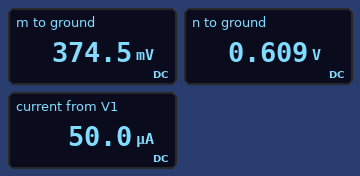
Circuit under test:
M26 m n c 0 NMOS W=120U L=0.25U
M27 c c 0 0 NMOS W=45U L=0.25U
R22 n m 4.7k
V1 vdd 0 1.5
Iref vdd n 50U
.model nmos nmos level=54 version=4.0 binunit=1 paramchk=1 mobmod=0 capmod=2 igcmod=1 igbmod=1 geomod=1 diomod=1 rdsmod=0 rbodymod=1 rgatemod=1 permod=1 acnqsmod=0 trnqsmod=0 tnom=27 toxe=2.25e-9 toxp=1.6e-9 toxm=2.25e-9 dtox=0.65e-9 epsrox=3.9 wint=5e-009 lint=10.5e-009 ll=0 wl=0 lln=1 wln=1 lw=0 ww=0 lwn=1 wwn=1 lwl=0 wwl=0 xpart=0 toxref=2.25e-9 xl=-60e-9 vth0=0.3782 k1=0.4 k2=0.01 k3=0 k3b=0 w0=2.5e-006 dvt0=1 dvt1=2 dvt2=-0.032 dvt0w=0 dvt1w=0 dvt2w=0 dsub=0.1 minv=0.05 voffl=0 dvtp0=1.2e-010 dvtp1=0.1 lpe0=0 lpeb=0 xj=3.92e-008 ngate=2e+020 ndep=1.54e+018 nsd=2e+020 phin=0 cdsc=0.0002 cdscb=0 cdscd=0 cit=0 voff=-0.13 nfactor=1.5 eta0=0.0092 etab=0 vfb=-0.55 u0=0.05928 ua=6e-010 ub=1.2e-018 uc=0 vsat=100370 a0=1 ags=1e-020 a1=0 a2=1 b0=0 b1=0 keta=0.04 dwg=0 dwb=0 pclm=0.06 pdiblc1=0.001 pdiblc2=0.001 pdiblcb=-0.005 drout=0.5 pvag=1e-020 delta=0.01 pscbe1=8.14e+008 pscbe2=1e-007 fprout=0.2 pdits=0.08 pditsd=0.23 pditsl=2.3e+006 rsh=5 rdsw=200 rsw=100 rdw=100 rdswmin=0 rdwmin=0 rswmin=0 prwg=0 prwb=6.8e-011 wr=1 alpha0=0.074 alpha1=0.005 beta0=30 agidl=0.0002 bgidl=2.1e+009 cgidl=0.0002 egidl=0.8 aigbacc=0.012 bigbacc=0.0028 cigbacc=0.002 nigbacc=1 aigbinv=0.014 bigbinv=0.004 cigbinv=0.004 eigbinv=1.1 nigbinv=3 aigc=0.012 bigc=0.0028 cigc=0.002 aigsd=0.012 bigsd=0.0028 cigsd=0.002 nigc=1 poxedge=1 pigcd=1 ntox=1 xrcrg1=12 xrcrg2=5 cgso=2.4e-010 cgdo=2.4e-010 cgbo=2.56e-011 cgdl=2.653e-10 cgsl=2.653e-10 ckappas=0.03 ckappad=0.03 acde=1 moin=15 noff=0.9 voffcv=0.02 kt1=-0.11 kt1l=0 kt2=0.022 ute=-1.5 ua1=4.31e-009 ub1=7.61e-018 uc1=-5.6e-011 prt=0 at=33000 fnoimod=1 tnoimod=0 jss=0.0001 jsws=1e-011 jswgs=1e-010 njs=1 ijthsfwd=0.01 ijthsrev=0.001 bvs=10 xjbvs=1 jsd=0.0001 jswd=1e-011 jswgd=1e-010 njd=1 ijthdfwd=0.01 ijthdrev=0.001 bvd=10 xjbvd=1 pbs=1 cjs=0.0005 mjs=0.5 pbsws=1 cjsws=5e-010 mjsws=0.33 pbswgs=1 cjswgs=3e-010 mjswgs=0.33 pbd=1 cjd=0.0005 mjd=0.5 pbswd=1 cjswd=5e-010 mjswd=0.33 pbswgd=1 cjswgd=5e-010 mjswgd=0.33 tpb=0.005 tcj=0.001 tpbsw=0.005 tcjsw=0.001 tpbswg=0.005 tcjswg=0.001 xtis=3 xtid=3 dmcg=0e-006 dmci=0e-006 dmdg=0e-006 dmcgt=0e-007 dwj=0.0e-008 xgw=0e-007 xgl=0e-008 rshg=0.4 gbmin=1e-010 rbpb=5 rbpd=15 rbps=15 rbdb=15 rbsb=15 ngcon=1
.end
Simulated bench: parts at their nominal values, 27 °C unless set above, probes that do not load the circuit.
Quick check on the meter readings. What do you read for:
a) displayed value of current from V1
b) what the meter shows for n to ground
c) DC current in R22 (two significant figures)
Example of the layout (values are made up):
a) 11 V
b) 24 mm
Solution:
a) 50.0 µA
b) 0.609 V
c) 50 µA
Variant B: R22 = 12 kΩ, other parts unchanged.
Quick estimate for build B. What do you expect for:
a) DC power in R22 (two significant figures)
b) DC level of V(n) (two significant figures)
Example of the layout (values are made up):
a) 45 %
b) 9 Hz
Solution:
a) 30 µW
b) 890 mV
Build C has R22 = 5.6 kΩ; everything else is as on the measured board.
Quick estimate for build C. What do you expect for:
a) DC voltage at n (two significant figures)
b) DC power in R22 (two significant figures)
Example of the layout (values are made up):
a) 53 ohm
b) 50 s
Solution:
a) 620 mV
b) 14 µW
